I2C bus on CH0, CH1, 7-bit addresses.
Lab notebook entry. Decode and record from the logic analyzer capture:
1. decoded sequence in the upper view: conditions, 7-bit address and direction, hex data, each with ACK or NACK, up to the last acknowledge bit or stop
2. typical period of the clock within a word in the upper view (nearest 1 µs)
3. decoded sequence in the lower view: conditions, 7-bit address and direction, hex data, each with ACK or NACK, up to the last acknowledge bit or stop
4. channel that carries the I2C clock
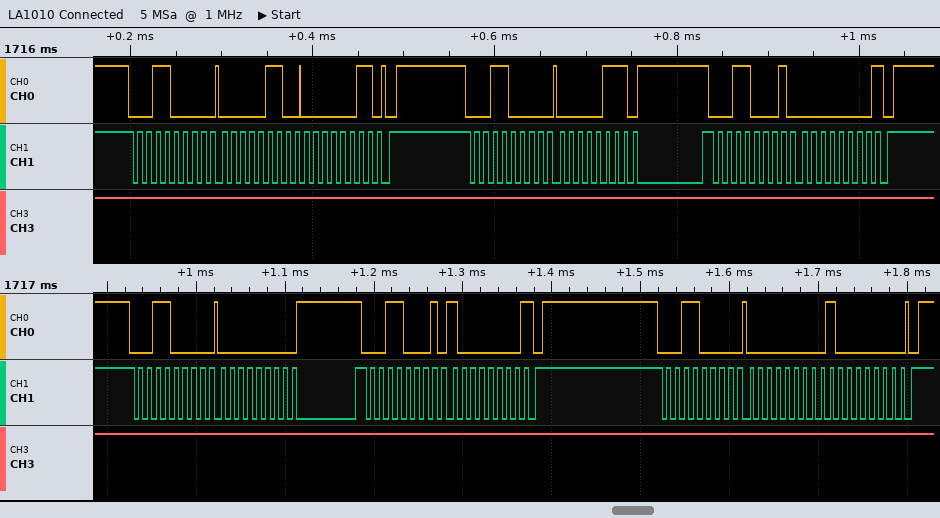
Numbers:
start, address 18 write ACK, 06 ACK, 03 ACK, stop, start, address 18 write ACK, 07 ACK, repeated start, address 18 read ACK, 00 NACK, stop
10 µs
start, address 18 write ACK, 00 ACK, repeated start, address 18 read ACK, 80 NACK, stop, start, address 18 write ACK, 00 ACK, 80 ACK, stop
CH1
